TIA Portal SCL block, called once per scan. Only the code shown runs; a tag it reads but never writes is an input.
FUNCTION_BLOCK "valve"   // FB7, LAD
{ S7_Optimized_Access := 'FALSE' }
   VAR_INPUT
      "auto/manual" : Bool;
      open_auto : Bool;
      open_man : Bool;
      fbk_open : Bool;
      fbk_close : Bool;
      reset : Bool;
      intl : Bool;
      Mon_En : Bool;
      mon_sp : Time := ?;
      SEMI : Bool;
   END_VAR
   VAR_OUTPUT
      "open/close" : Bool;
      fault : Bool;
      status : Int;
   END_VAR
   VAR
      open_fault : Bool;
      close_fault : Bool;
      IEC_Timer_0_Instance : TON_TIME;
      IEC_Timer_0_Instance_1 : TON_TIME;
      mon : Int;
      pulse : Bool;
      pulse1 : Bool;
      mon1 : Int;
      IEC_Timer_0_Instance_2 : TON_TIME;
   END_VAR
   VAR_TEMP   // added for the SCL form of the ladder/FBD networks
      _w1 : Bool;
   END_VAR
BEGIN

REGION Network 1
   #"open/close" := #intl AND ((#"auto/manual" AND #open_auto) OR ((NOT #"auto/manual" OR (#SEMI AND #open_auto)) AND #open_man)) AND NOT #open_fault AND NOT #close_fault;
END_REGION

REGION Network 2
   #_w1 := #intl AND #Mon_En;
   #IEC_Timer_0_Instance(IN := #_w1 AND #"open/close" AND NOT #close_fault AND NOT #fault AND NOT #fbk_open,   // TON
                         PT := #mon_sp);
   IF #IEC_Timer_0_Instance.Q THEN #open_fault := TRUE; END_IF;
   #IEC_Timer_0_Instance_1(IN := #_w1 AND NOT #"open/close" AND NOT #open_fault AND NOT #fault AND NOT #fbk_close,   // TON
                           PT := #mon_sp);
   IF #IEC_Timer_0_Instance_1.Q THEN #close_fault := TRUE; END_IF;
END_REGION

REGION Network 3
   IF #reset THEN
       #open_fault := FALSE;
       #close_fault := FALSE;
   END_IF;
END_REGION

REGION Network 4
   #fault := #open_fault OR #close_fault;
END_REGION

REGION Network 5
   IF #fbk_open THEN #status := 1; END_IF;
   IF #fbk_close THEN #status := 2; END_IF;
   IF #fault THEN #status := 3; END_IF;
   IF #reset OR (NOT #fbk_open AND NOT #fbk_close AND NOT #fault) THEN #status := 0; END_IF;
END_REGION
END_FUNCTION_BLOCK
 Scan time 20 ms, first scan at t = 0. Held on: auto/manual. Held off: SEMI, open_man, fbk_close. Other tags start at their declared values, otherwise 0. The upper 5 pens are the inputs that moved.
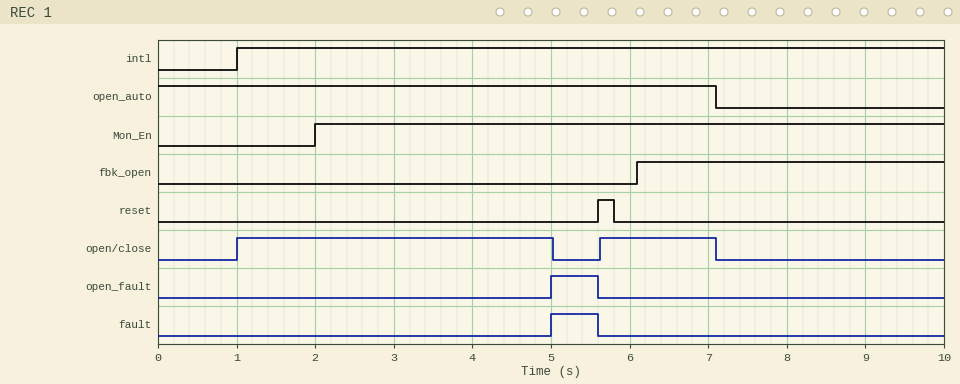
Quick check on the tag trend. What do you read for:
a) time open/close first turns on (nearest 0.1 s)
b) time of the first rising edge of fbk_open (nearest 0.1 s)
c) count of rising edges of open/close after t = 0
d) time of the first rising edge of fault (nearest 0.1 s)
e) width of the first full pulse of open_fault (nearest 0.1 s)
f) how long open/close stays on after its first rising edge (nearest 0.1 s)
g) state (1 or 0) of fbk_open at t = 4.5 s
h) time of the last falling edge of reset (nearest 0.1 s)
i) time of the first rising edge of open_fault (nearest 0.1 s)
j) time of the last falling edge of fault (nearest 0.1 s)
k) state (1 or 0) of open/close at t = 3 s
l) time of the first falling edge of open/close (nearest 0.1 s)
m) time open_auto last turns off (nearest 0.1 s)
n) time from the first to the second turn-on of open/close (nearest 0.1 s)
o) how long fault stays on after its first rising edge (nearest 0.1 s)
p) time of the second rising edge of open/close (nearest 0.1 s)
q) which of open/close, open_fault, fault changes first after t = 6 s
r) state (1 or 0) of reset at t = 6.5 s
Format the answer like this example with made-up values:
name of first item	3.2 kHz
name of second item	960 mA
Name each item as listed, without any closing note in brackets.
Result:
time open/close first turns on	1.0 s
time of the first rising edge of fbk_open	6.1 s
count of rising edges of open/close after t = 0	2
time of the first rising edge of fault	5.0 s
width of the first full pulse of open_fault	0.6 s
how long open/close stays on after its first rising edge	4.0 s
state (1 or 0) of fbk_open at t = 4.5 s	0
time of the last falling edge of reset	5.8 s
time of the first rising edge of open_fault	5.0 s
time of the last falling edge of fault	5.6 s
state (1 or 0) of open/close at t = 3 s	1
time of the first falling edge of open/close	5.0 s
time open_auto last turns off	7.1 s
time from the first to the second turn-on of open/close	4.6 s
how long fault stays on after its first rising edge	0.6 s
time of the second rising edge of open/close	5.6 s
which of open/close, open_fault, fault changes first after t = 6 s	open/close
state (1 or 0) of reset at t = 6.5 s	0
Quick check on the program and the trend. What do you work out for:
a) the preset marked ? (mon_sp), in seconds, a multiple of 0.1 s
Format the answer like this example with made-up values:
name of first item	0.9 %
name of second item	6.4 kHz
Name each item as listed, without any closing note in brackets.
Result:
the preset marked ? (mon_sp), in seconds, a multiple of 0.1 s	3.0 s
